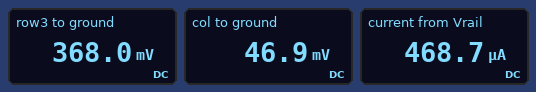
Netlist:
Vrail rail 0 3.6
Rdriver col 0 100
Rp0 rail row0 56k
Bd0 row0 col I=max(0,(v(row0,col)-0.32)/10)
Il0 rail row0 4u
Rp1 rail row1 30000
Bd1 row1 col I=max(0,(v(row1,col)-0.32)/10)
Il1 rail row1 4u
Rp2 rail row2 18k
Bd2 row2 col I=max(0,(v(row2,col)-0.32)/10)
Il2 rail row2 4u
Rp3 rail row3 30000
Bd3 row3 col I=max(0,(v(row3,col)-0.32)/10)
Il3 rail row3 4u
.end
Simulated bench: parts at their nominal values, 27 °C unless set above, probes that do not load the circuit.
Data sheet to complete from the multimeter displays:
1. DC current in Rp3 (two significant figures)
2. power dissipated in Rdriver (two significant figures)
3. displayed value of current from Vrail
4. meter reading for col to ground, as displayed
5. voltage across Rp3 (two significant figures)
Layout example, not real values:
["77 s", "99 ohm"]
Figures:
["110 µA", "22 µW", "468.7 µA", "46.9 mV", "3.2 V"]
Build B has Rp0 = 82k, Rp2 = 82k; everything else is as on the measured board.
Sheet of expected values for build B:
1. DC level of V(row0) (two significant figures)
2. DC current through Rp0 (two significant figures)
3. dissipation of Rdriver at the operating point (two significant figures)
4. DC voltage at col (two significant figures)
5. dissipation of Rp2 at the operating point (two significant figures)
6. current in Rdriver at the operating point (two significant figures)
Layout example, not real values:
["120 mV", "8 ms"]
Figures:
["350 mV", "40 µA", "9.7 µW", "31 mV", "130 µW", "310 µA"]
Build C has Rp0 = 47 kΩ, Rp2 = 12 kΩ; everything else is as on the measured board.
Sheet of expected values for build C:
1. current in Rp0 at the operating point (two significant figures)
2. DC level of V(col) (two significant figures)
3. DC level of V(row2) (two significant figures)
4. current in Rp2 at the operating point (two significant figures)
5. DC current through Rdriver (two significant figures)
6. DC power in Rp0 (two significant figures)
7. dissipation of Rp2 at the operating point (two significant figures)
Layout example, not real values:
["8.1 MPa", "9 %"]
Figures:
["69 µA", "57 mV", "380 mV", "270 µA", "570 µA", "220 µW", "860 µW"]
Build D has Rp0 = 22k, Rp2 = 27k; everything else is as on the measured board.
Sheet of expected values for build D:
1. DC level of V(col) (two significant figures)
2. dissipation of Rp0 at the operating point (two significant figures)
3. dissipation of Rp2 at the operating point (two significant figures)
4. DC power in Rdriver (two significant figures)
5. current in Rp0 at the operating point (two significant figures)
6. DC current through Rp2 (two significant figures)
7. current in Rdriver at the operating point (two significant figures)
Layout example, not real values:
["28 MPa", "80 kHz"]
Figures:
["50 mV", "470 µW", "390 µW", "25 µW", "150 µA", "120 µA", "500 µA"]
